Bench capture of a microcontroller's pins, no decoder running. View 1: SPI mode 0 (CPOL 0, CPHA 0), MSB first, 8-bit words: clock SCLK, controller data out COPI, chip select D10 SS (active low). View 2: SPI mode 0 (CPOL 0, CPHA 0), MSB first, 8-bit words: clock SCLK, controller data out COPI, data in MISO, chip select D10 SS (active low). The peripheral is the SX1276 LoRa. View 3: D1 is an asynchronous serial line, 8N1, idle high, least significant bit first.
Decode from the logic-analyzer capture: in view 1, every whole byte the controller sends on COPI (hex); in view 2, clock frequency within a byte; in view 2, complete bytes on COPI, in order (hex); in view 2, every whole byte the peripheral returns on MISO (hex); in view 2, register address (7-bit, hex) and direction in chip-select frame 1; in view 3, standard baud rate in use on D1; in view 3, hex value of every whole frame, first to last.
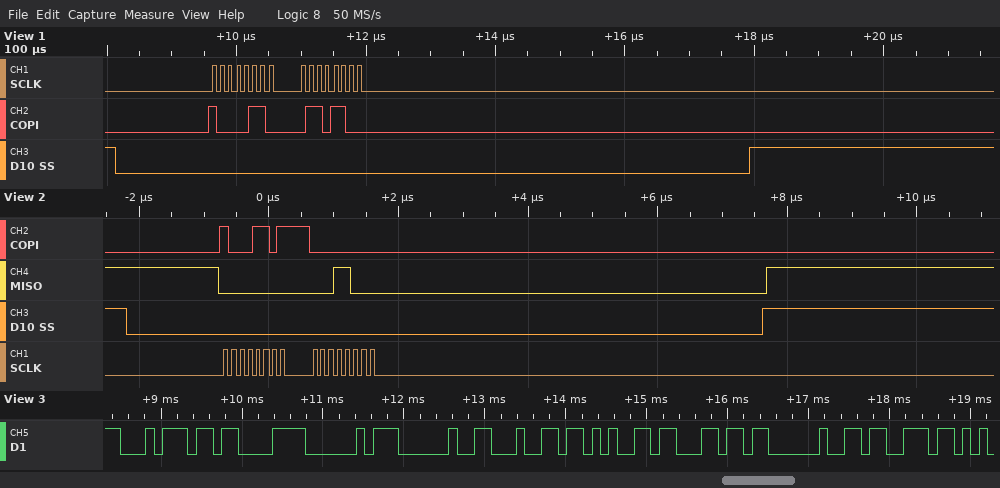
86 6C
8 MHz
8D 00
00 18
0x0D write
9600 baud
74 C3 A0 20 64 65 6C 20 73
